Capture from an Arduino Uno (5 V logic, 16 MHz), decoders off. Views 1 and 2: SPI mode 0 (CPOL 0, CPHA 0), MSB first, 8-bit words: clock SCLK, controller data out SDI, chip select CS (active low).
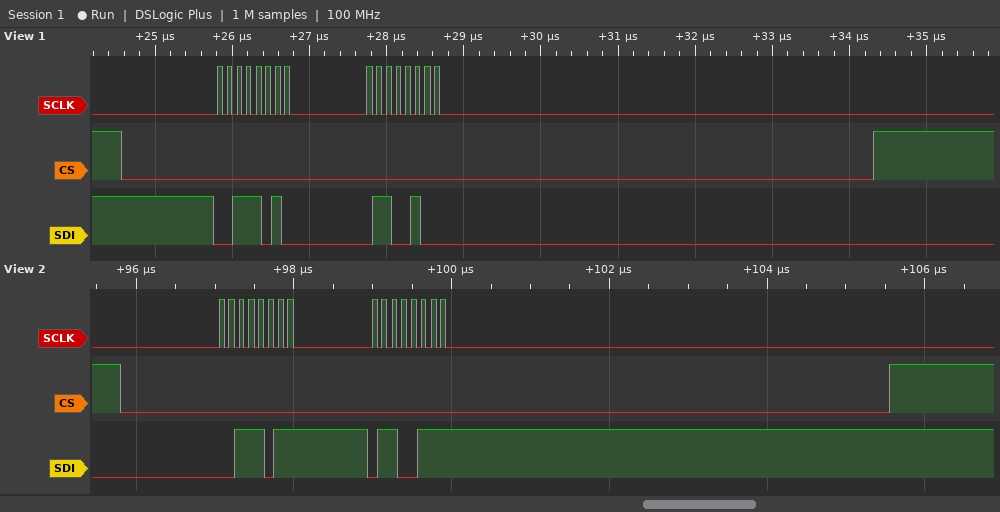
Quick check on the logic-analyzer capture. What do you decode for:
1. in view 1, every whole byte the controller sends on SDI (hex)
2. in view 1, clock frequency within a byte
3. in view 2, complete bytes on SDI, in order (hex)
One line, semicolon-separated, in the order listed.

3A 64; 8 MHz; 3B 67
